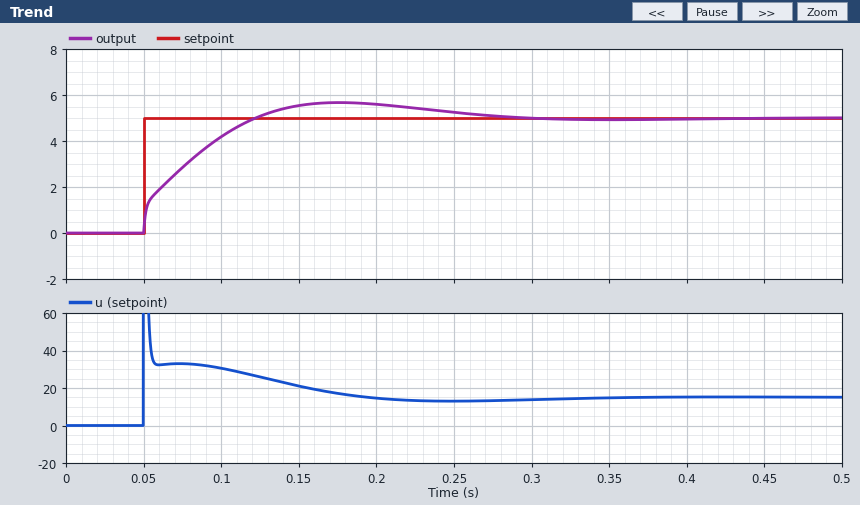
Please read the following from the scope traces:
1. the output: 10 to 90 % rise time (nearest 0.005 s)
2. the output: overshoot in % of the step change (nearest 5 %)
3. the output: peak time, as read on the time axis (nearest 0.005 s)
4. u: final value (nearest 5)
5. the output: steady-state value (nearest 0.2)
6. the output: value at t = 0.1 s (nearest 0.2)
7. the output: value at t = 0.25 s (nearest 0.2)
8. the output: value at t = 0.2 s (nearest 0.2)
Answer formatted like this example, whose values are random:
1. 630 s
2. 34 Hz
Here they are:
1. 0.055 s
2. 15 %
3. 0.175 s
4. 15
5. 5.0
6. 4.2
7. 5.2
8. 5.6
